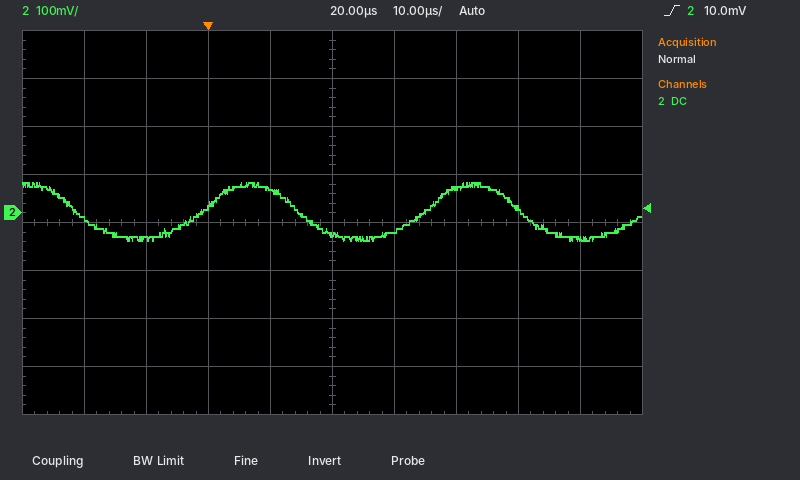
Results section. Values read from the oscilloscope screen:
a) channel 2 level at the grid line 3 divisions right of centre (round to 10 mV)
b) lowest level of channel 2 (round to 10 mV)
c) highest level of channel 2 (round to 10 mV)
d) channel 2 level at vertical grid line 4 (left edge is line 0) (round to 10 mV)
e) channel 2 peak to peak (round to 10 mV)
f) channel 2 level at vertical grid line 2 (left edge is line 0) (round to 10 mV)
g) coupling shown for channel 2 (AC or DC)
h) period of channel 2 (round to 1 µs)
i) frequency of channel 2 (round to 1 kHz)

10 mV
-60 mV
60 mV
50 mV
120 mV
-50 mV
DC
36 µs
28 kHz
